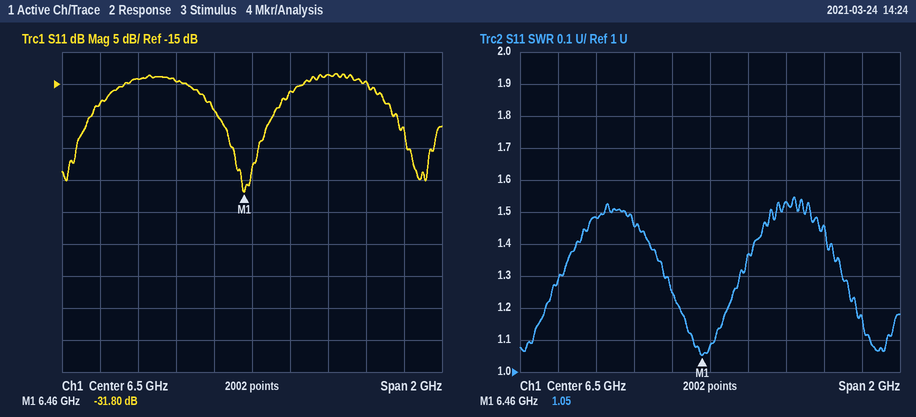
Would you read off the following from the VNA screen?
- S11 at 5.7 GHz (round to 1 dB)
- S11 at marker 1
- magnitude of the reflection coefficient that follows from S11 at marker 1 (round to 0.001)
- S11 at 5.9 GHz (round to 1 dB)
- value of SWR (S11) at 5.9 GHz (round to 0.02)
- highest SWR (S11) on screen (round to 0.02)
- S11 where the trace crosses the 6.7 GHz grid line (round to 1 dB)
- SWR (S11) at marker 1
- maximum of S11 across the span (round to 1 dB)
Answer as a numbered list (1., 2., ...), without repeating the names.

1. -18 dB
2. -31.80 dB
3. 0.026
4. -14 dB
5. 1.48
6. 1.54
7. -16 dB
8. 1.05
9. -13 dB
